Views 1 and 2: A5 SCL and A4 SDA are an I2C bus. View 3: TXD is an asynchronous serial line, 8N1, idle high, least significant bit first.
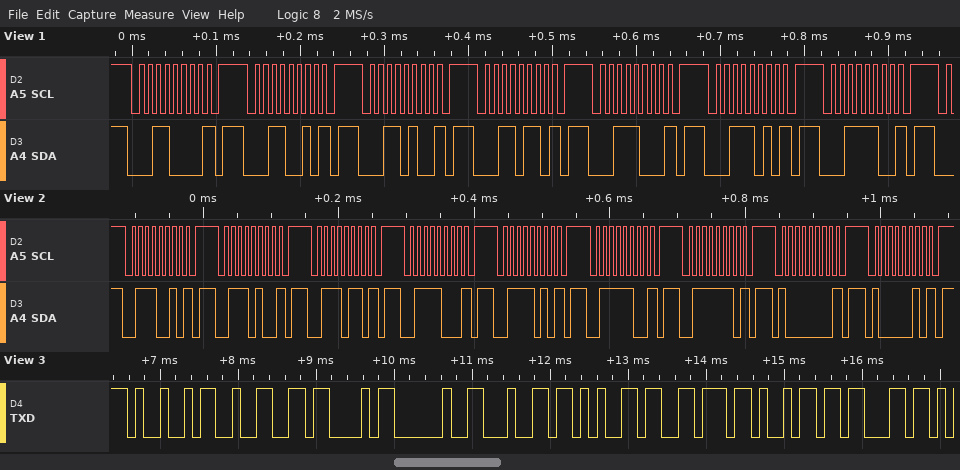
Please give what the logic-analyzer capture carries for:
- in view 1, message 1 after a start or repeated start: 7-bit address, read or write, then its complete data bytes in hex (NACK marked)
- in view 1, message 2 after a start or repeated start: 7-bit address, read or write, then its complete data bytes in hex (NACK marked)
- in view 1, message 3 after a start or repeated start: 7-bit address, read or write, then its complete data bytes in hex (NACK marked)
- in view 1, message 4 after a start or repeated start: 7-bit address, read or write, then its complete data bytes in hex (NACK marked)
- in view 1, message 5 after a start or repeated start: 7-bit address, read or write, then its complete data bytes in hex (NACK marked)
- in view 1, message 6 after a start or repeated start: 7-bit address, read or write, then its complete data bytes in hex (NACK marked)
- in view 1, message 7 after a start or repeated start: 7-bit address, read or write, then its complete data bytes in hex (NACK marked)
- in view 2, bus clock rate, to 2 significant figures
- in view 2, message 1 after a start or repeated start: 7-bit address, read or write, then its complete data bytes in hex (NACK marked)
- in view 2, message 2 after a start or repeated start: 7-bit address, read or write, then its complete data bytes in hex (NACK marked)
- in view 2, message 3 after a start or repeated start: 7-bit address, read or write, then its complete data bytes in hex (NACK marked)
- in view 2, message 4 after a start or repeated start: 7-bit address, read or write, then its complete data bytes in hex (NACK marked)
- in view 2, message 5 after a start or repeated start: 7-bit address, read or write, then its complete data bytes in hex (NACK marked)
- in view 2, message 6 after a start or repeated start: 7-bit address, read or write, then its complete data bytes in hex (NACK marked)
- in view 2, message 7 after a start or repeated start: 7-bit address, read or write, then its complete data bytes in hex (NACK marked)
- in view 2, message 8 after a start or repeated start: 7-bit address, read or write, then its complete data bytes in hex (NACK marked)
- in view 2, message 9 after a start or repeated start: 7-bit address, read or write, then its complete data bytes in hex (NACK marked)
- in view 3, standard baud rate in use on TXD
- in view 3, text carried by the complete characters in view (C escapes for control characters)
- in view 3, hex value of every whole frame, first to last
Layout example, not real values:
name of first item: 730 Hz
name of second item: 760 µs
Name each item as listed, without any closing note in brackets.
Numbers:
in view 1, message 1 after a start or repeated start: 7-bit address, read or write, then its complete data bytes in hex: 0x18 write NACK
in view 1, message 2 after a start or repeated start: 7-bit address, read or write, then its complete data bytes in hex: 0x19 write NACK
in view 1, message 3 after a start or repeated start: 7-bit address, read or write, then its complete data bytes in hex: 0x1A write NACK
in view 1, message 4 after a start or repeated start: 7-bit address, read or write, then its complete data bytes in hex: 0x1B write NACK
in view 1, message 5 after a start or repeated start: 7-bit address, read or write, then its complete data bytes in hex: 0x1C write NACK
in view 1, message 6 after a start or repeated start: 7-bit address, read or write, then its complete data bytes in hex: 0x1D write NACK
in view 1, message 7 after a start or repeated start: 7-bit address, read or write, then its complete data bytes in hex: 0x1E write NACK
in view 2, bus clock rate, to 2 significant figures: 100 kHz
in view 2, message 1 after a start or repeated start: 7-bit address, read or write, then its complete data bytes in hex: 0x39 write NACK
in view 2, message 2 after a start or repeated start: 7-bit address, read or write, then its complete data bytes in hex: 0x3A write NACK
in view 2, message 3 after a start or repeated start: 7-bit address, read or write, then its complete data bytes in hex: 0x3B write NACK
in view 2, message 4 after a start or repeated start: 7-bit address, read or write, then its complete data bytes in hex: 0x3C write NACK
in view 2, message 5 after a start or repeated start: 7-bit address, read or write, then its complete data bytes in hex: 0x3D write NACK
in view 2, message 6 after a start or repeated start: 7-bit address, read or write, then its complete data bytes in hex: 0x3E write NACK
in view 2, message 7 after a start or repeated start: 7-bit address, read or write, then its complete data bytes in hex: 0x3F write NACK
in view 2, message 8 after a start or repeated start: 7-bit address, read or write, then its complete data bytes in hex: 0x40 write NACK
in view 2, message 9 after a start or repeated start: 7-bit address, read or write, then its complete data bytes in hex: 0x41 write NACK
in view 3, standard baud rate in use on TXD: 9600 baud
in view 3, text carried by the complete characters in view: "I2C devic"
in view 3, hex value of every whole frame, first to last: 0x49 0x32 0x43 0x20 0x64 0x65 0x76 0x69 0x63
